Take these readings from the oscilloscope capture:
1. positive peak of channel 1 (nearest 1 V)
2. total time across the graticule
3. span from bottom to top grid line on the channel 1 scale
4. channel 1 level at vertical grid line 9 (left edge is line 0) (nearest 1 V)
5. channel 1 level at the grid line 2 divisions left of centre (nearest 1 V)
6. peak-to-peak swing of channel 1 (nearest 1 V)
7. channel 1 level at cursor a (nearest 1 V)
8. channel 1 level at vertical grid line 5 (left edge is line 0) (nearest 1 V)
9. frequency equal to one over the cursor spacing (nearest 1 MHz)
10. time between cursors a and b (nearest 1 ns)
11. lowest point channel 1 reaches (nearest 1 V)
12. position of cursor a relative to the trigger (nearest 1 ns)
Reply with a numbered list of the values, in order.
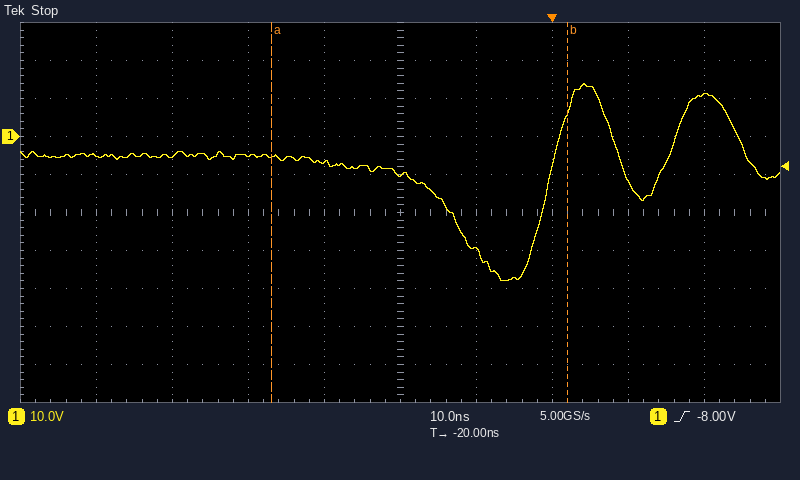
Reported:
1. 14 V
2. 100 ns
3. 100 V
4. 11 V
5. -5 V
6. 52 V
7. -5 V
8. -10 V
9. 26 MHz
10. 39 ns
11. -38 V
12. -37 ns
